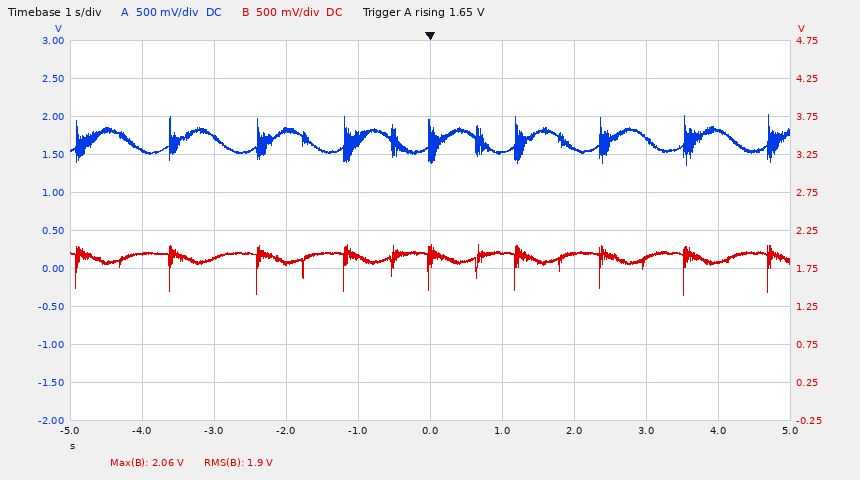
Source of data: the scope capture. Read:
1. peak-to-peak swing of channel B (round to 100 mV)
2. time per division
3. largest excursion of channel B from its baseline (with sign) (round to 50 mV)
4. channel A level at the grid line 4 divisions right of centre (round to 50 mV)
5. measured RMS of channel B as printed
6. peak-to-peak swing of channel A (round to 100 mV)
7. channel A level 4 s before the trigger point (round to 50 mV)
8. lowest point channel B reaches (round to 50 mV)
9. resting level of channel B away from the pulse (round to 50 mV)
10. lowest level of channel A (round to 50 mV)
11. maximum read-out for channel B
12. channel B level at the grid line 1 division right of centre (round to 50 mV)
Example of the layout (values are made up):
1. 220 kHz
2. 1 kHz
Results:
1. 700 mV
2. 1 s
3. -550 mV
4. 1.80 V
5. 1.9 V
6. 700 mV
7. 1.55 V
8. 1.40 V
9. 1.95 V
10. 1.35 V
11. 2.06 V
12. 1.95 V
